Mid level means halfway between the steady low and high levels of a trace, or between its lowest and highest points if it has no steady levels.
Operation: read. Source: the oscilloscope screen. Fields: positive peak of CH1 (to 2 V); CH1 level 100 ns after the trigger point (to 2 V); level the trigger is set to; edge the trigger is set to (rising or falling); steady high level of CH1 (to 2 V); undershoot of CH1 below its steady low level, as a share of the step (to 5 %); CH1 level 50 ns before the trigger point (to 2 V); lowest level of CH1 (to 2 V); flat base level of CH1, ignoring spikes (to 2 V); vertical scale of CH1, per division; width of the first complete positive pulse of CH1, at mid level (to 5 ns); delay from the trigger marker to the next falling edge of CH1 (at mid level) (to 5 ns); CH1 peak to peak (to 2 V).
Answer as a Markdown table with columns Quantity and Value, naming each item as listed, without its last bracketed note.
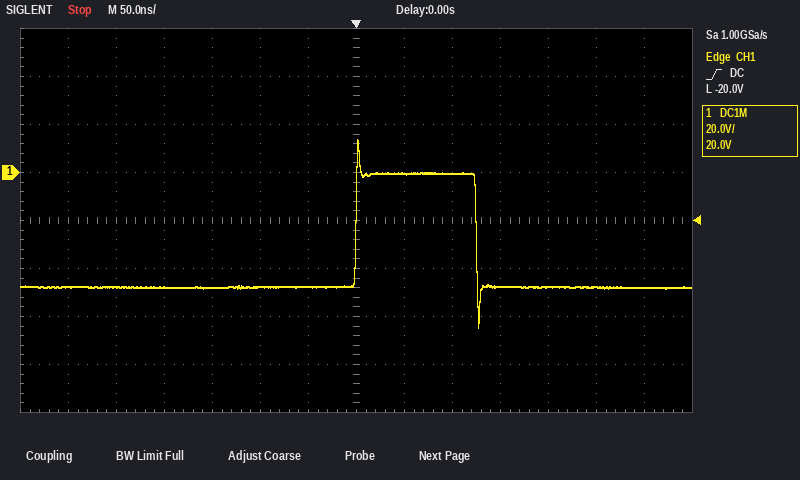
| Quantity | Value |
|---|---|
| positive peak of CH1 | 14 V |
| CH1 level 100 ns after the trigger point | 0 V |
| level the trigger is set to | -20.0 V |
| edge the trigger is set to | rising |
| steady high level of CH1 | 0 V |
| undershoot of CH1 below its steady low level, as a share of the step | 35 % |
| CH1 level 50 ns before the trigger point | -48 V |
| lowest level of CH1 | -64 V |
| flat base level of CH1, ignoring spikes | -48 V |
| vertical scale of CH1, per division | 20 V |
| width of the first complete positive pulse of CH1, at mid level | 125 ns |
| delay from the trigger marker to the next falling edge of CH1 (at mid level) | 125 ns |
| CH1 peak to peak | 78 V |
